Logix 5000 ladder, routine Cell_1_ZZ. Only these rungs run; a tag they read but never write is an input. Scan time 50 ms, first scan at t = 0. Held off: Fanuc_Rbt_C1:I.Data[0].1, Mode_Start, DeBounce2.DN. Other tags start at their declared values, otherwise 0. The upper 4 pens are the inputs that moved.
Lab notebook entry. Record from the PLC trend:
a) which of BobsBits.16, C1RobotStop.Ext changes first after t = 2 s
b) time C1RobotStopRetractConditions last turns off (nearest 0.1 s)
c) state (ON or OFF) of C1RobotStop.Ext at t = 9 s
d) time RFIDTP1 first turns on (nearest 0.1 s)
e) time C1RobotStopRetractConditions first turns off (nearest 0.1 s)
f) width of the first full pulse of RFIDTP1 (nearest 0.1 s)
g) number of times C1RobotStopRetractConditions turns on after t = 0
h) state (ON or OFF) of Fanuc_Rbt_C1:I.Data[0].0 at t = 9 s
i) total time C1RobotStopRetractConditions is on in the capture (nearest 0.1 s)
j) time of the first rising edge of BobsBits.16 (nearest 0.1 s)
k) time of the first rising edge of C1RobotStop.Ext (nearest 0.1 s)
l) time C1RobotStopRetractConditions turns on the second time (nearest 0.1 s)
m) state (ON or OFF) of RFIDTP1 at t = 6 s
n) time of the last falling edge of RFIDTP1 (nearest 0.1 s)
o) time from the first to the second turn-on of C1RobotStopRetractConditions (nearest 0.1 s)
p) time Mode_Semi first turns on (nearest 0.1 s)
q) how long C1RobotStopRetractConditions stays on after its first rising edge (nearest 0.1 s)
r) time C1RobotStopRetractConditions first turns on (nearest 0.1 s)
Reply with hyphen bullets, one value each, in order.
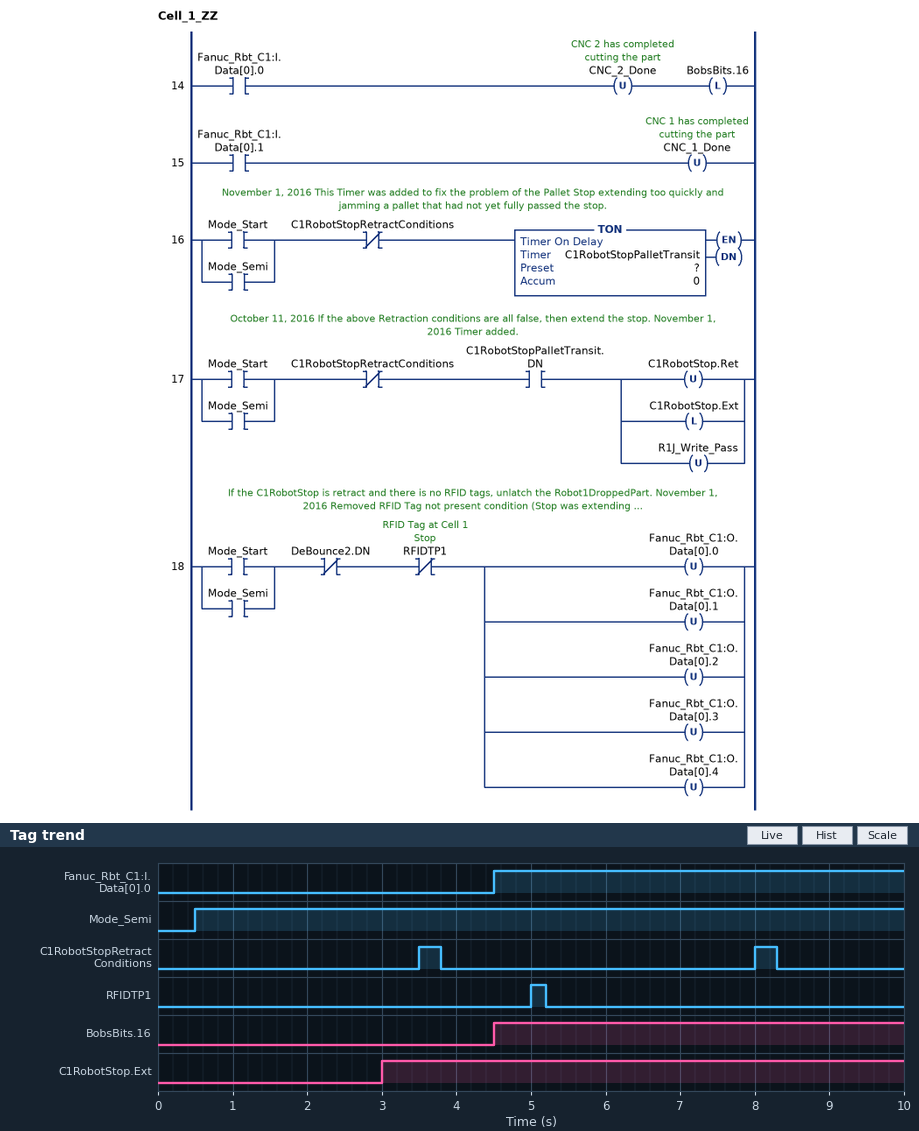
- C1RobotStop.Ext
- 8.3 s
- ON
- 5.0 s
- 3.8 s
- 0.2 s
- 2
- ON
- 0.6 s
- 4.5 s
- 3.0 s
- 8.0 s
- OFF
- 5.2 s
- 4.5 s
- 0.5 s
- 0.3 s
- 3.5 s
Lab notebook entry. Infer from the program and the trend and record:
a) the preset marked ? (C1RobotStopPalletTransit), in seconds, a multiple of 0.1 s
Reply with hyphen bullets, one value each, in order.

- 2.5 s
